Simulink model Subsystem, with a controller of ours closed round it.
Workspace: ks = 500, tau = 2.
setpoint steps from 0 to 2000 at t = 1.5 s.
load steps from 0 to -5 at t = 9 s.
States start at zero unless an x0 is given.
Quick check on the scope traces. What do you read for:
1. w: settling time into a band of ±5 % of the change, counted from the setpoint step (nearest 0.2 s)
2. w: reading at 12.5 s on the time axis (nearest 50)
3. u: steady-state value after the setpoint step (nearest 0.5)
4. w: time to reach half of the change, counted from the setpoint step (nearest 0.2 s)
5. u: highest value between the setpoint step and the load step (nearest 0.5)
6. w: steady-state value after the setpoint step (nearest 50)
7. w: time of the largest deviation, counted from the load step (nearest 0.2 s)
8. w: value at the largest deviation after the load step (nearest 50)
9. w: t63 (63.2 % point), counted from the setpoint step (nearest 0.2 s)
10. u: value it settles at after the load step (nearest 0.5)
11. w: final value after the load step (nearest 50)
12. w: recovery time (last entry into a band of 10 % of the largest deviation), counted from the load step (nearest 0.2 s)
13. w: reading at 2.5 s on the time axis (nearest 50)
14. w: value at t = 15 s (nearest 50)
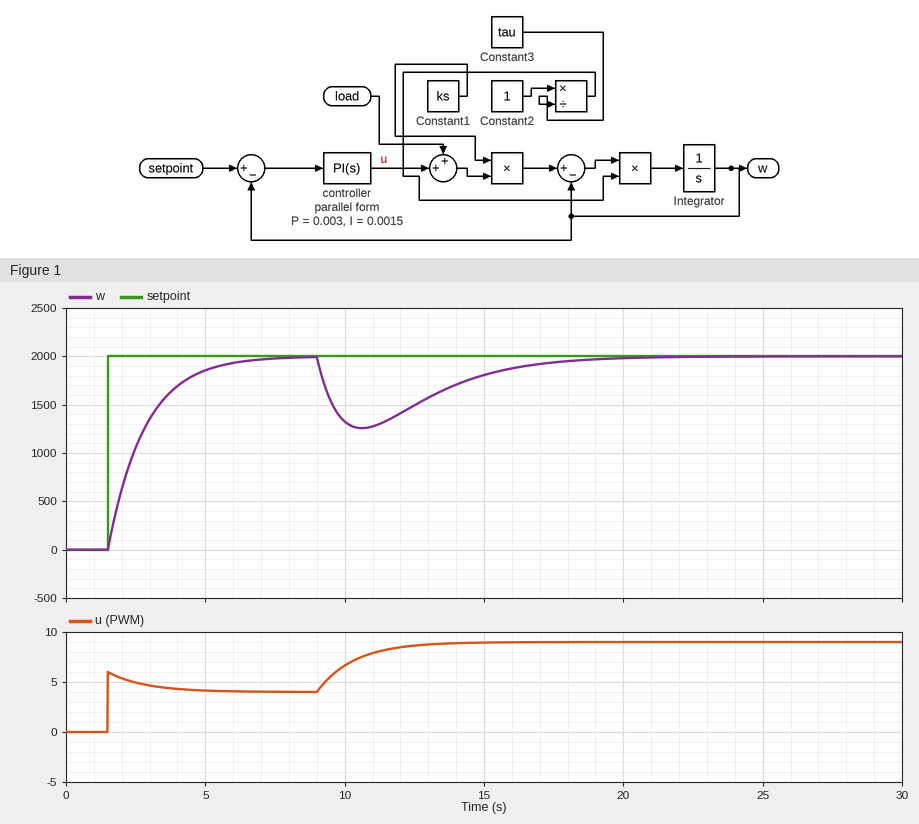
4.0 s
1500
4.0
1.0 s
6.0
2000
1.6 s
1250
1.4 s
9.0
2000
8.2 s
1050
1800
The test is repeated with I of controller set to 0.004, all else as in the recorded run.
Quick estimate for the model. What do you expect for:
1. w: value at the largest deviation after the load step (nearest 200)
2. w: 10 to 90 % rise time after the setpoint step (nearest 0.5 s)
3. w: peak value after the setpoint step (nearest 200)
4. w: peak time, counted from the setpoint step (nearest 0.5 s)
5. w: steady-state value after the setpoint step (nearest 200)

1400
1.5 s
2200
3.0 s
2000
